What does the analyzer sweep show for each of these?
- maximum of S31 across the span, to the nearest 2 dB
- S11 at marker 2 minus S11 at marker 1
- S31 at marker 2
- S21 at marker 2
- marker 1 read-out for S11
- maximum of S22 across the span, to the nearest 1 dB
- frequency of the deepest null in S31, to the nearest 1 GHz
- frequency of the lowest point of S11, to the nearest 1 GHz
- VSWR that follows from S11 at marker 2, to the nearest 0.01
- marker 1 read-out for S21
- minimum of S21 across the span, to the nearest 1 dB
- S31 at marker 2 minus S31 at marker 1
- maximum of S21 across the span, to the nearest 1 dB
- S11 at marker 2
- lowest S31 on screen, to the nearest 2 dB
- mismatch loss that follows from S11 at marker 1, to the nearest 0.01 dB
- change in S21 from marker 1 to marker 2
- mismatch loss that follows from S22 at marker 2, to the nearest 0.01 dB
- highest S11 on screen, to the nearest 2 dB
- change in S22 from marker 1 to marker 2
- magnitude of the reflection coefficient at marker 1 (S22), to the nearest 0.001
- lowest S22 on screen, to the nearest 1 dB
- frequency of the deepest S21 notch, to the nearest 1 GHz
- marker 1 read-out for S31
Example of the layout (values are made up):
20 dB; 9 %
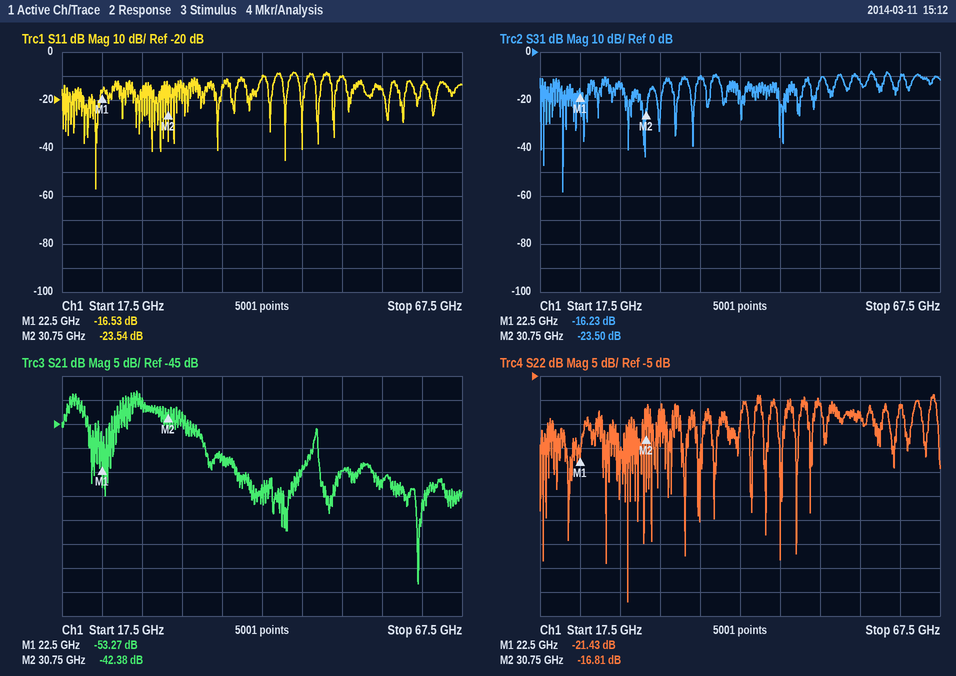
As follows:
-8 dB; -7.01 dB; -23.50 dB; -42.38 dB; -16.53 dB; -9 dB; 20 GHz; 22 GHz; 1.14; -53.27 dB; -78 dB; -7.27 dB; -38 dB; -23.54 dB; -58 dB; 0.10 dB; 10.89 dB; 0.09 dB; -8 dB; 4.62 dB; 0.085; -52 dB; 62 GHz; -16.23 dB
